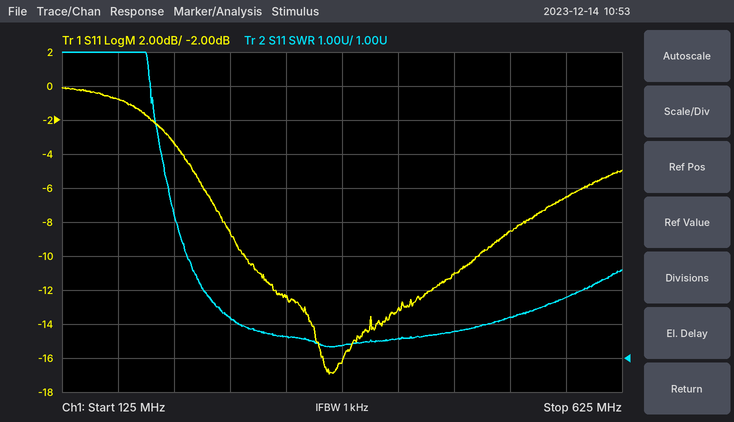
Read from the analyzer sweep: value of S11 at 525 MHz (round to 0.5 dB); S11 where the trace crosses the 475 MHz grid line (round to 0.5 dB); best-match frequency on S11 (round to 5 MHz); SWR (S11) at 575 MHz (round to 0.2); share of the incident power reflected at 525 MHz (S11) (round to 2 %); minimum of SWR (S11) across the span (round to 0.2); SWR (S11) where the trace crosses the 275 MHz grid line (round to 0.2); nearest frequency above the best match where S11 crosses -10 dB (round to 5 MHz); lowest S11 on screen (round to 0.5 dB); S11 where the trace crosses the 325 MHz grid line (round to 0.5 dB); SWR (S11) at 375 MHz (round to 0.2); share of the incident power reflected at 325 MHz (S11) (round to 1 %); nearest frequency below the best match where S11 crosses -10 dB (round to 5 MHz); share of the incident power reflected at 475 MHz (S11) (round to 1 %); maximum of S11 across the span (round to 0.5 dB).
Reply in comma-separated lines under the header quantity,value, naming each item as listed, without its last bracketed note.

quantity,value
value of S11 at 525 MHz,-8.5 dB
S11 where the trace crosses the 475 MHz grid line,-11.0 dB
best-match frequency on S11,365 MHz
SWR (S11) at 575 MHz,2.8
share of the incident power reflected at 525 MHz (S11),14 %
minimum of SWR (S11) across the span,1.4
SWR (S11) where the trace crosses the 275 MHz grid line,2.2
nearest frequency above the best match where S11 crosses -10 dB,495 MHz
lowest S11 on screen,-17.0 dB
S11 where the trace crosses the 325 MHz grid line,-12.5 dB
SWR (S11) at 375 MHz,1.4
share of the incident power reflected at 325 MHz (S11),6 %
nearest frequency below the best match where S11 crosses -10 dB,290 MHz
share of the incident power reflected at 475 MHz (S11),8 %
maximum of S11 across the span,0.0 dB
